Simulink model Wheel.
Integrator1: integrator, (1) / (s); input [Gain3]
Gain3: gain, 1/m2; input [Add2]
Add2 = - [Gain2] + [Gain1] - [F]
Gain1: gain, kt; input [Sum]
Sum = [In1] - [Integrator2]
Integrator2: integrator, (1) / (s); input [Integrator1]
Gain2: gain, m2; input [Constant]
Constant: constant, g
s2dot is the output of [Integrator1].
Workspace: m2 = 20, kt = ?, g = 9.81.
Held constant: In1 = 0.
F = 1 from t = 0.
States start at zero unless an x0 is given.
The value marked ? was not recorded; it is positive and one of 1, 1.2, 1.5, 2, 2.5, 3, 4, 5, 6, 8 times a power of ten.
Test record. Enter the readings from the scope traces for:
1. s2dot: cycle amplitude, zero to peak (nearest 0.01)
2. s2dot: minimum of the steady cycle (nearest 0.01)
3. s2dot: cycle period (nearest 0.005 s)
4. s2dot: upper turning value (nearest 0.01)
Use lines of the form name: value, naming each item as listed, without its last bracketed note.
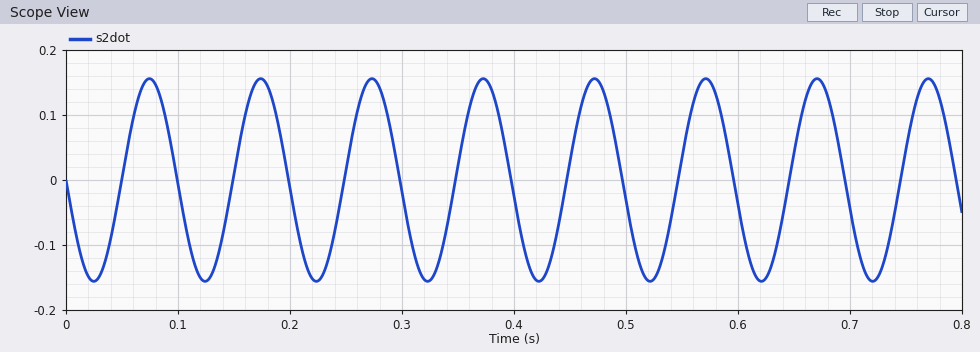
s2dot: cycle amplitude, zero to peak: 0.16
s2dot: minimum of the steady cycle: -0.16
s2dot: cycle period: 0.100 s
s2dot: upper turning value: 0.16
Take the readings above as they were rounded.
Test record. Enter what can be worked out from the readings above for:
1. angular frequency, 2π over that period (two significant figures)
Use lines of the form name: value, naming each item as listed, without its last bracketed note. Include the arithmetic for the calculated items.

angular frequency, 2π over that period: 2π / 0.1 = 63 rad/s
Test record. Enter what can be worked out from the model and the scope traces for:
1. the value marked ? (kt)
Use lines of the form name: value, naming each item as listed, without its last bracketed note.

the value marked ?: 80000
